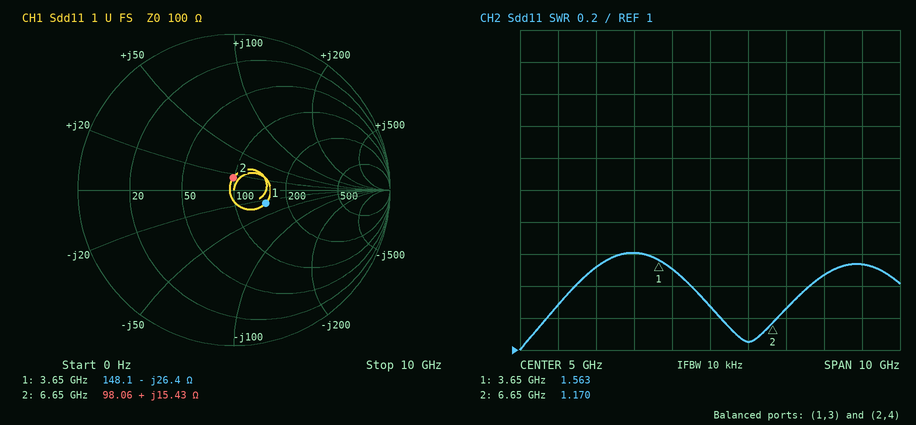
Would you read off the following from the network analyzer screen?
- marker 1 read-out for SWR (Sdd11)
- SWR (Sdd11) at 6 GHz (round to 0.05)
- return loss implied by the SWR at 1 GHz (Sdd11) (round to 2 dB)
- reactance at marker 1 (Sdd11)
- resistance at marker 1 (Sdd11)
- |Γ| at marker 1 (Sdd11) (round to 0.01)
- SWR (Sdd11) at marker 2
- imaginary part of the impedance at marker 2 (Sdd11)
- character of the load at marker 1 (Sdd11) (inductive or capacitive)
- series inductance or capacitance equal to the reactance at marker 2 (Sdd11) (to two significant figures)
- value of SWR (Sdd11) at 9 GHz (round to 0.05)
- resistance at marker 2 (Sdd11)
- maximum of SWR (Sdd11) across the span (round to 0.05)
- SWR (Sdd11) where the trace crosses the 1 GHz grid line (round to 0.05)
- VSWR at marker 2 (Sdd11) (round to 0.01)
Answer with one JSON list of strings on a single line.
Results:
["1.563", "1.05", "18 dB", "-26.4 Ω", "148.1 Ω", "0.22", "1.170", "+15.43 Ω", "capacitive", "370 pH", "1.55", "98.06 Ω", "1.60", "1.30", "1.17"]
